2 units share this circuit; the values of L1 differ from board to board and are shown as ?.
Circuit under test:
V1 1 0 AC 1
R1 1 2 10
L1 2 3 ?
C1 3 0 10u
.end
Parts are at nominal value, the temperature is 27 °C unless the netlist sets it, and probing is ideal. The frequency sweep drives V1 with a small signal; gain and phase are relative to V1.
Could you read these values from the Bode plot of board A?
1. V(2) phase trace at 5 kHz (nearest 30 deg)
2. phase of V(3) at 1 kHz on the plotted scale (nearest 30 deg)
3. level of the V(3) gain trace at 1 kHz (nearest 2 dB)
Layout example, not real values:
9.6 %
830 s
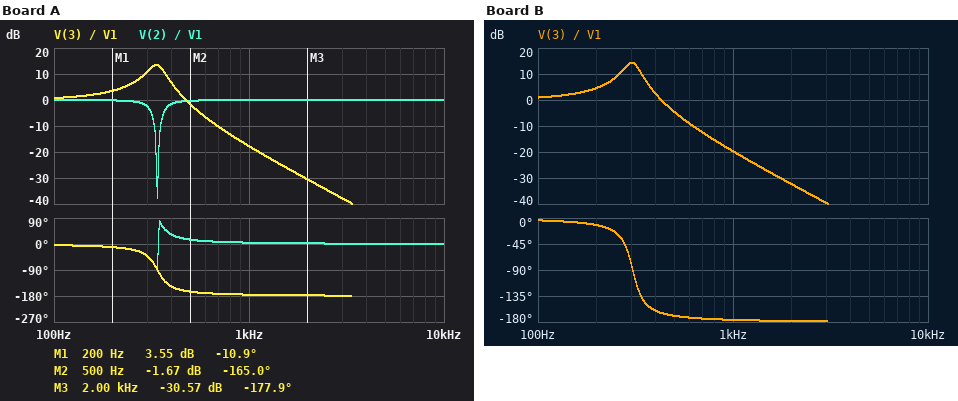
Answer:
0 deg
-180 deg
-18 dB
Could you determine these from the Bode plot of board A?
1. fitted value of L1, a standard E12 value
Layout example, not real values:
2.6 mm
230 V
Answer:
22 mH
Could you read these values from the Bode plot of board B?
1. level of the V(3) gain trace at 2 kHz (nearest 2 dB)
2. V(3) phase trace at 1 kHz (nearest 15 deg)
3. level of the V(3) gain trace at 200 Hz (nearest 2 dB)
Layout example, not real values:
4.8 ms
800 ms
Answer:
-32 dB
-180 deg
4 dB
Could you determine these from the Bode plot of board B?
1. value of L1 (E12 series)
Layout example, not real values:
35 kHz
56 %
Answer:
27 mH
